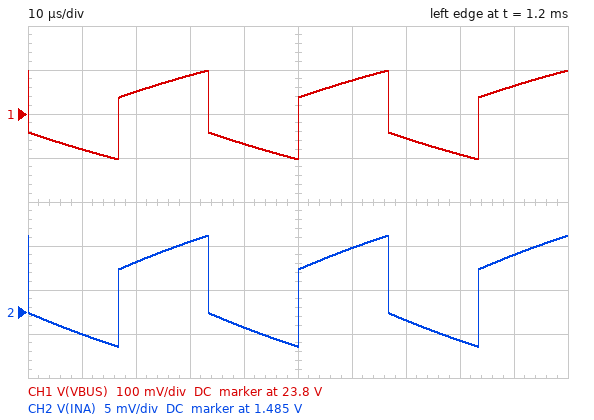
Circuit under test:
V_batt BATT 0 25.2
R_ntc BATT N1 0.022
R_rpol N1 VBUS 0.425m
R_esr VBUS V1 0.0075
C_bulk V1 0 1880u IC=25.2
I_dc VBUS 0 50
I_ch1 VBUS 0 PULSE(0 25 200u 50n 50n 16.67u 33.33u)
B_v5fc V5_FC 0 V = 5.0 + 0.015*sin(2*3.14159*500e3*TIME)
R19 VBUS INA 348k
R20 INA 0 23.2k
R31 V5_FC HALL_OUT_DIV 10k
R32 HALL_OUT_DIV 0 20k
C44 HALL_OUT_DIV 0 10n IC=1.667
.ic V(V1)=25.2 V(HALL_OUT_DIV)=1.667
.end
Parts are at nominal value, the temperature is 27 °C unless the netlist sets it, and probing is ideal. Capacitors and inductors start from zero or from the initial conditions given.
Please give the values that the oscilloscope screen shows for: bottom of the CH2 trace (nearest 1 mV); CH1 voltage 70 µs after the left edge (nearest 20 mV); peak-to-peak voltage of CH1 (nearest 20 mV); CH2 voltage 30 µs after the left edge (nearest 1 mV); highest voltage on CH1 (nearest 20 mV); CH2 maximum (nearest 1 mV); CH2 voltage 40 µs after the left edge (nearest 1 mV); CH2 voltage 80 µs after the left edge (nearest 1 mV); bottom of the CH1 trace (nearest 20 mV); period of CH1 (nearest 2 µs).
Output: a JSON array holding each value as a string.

["1.481 V", "23.74 V", "200 mV", "1.493 V", "23.90 V", "1.494 V", "1.483 V", "1.482 V", "23.70 V", "34 µs"]
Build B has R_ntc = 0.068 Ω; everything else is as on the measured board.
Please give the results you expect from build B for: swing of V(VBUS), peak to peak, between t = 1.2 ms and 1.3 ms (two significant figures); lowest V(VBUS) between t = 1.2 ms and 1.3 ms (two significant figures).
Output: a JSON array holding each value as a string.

["260 mV", "21 V"]
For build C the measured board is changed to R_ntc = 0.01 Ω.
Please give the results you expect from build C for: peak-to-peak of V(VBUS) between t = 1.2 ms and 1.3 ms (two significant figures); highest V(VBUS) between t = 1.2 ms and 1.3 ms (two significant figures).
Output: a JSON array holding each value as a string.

["150 mV", "25 V"]
